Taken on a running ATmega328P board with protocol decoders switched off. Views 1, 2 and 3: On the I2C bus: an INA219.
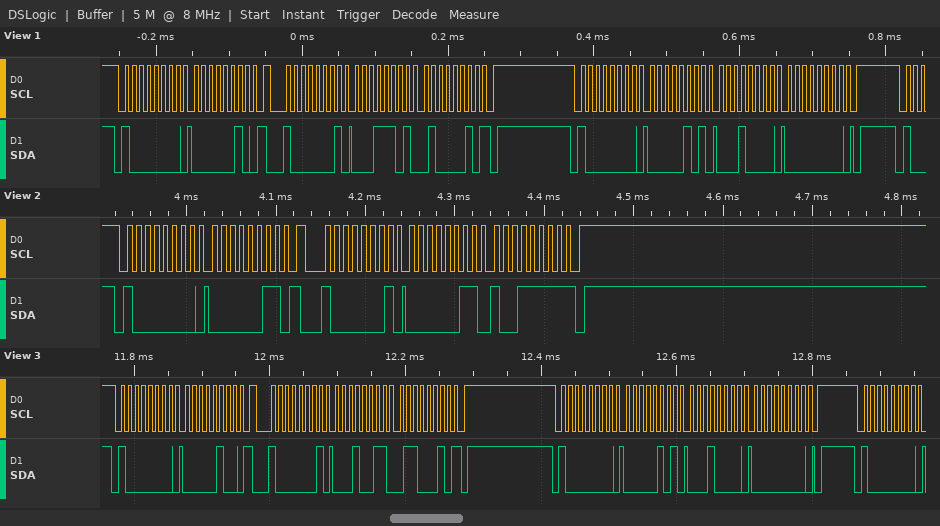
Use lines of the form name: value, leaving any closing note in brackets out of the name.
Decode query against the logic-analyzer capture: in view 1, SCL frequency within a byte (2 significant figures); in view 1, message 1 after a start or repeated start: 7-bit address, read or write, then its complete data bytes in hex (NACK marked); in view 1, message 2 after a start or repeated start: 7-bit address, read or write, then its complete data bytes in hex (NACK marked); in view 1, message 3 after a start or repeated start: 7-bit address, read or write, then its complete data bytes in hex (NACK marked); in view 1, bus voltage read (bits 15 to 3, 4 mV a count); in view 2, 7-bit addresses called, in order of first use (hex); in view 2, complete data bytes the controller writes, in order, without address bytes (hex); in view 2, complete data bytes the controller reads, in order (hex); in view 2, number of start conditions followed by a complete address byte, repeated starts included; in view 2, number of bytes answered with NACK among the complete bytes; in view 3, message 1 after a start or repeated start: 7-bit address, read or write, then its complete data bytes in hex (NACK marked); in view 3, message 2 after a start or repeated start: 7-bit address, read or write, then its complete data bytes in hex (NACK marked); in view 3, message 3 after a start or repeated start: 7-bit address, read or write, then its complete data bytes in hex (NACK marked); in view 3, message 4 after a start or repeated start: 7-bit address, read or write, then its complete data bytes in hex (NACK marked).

in view 1, SCL frequency within a byte: 100 kHz
in view 1, message 1 after a start or repeated start: 7-bit address, read or write, then its complete data bytes in hex: 0x40 write: 02
in view 1, message 2 after a start or repeated start: 7-bit address, read or write, then its complete data bytes in hex: 0x40 read: 1D 42 NACK
in view 1, message 3 after a start or repeated start: 7-bit address, read or write, then its complete data bytes in hex: 0x40 write: 05 10 00
in view 1, bus voltage read: 3.744 V
in view 2, 7-bit addresses called, in order of first use: 0x40
in view 2, complete data bytes the controller writes, in order, without address bytes: 03
in view 2, complete data bytes the controller reads, in order: 03 9F
in view 2, number of start conditions followed by a complete address byte, repeated starts included: 2
in view 2, number of bytes answered with NACK among the complete bytes: 1
in view 3, message 1 after a start or repeated start: 7-bit address, read or write, then its complete data bytes in hex: 0x40 write: 04
in view 3, message 2 after a start or repeated start: 7-bit address, read or write, then its complete data bytes in hex: 0x40 read: 13 62 NACK
in view 3, message 3 after a start or repeated start: 7-bit address, read or write, then its complete data bytes in hex: 0x40 write: 05 10 00
in view 3, message 4 after a start or repeated start: 7-bit address, read or write, then its complete data bytes in hex: 0x40 write
